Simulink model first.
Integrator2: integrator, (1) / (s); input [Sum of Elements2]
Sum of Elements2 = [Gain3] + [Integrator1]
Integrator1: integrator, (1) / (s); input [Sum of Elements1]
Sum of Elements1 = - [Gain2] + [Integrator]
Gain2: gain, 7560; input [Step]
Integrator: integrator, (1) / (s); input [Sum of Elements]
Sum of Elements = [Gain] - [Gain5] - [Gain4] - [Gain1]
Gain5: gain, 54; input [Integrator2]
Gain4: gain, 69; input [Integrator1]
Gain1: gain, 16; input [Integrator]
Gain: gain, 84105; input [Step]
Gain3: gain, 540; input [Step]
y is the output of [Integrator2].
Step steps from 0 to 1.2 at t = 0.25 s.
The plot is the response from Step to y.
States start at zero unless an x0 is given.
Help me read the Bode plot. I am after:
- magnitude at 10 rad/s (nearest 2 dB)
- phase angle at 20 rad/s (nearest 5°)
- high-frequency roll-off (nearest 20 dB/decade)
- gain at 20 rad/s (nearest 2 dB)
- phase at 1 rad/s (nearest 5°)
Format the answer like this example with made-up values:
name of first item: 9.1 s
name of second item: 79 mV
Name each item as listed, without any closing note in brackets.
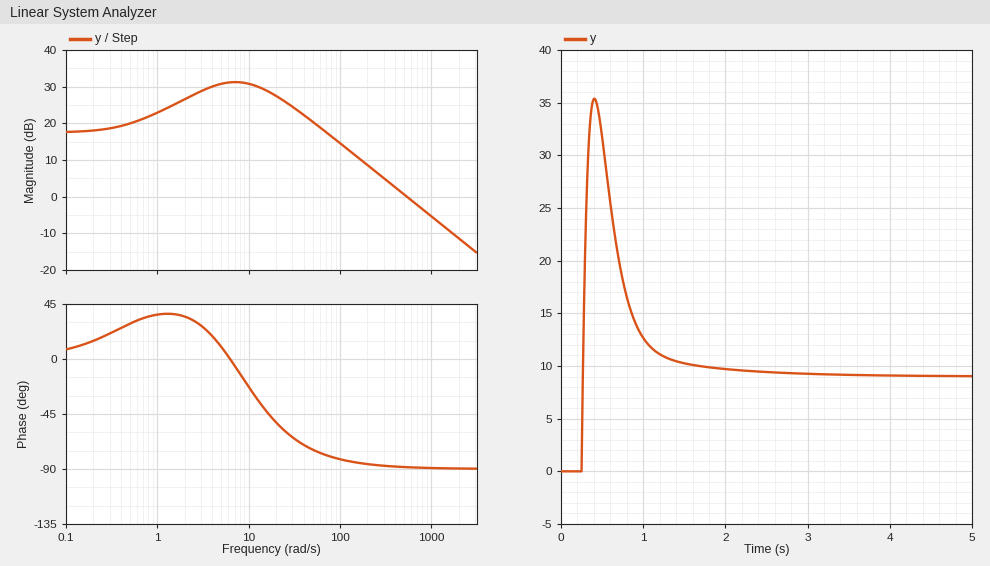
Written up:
magnitude at 10 rad/s: 30 dB
phase angle at 20 rad/s: -50°
high-frequency roll-off: -20 dB/decade
gain at 20 rad/s: 28 dB
phase at 1 rad/s: 35°
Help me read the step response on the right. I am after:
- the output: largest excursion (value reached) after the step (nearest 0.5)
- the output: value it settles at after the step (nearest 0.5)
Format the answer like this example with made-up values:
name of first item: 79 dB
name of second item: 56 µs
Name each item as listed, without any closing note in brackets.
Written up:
the output: largest excursion (value reached) after the step: 35.5
the output: value it settles at after the step: 9.0
